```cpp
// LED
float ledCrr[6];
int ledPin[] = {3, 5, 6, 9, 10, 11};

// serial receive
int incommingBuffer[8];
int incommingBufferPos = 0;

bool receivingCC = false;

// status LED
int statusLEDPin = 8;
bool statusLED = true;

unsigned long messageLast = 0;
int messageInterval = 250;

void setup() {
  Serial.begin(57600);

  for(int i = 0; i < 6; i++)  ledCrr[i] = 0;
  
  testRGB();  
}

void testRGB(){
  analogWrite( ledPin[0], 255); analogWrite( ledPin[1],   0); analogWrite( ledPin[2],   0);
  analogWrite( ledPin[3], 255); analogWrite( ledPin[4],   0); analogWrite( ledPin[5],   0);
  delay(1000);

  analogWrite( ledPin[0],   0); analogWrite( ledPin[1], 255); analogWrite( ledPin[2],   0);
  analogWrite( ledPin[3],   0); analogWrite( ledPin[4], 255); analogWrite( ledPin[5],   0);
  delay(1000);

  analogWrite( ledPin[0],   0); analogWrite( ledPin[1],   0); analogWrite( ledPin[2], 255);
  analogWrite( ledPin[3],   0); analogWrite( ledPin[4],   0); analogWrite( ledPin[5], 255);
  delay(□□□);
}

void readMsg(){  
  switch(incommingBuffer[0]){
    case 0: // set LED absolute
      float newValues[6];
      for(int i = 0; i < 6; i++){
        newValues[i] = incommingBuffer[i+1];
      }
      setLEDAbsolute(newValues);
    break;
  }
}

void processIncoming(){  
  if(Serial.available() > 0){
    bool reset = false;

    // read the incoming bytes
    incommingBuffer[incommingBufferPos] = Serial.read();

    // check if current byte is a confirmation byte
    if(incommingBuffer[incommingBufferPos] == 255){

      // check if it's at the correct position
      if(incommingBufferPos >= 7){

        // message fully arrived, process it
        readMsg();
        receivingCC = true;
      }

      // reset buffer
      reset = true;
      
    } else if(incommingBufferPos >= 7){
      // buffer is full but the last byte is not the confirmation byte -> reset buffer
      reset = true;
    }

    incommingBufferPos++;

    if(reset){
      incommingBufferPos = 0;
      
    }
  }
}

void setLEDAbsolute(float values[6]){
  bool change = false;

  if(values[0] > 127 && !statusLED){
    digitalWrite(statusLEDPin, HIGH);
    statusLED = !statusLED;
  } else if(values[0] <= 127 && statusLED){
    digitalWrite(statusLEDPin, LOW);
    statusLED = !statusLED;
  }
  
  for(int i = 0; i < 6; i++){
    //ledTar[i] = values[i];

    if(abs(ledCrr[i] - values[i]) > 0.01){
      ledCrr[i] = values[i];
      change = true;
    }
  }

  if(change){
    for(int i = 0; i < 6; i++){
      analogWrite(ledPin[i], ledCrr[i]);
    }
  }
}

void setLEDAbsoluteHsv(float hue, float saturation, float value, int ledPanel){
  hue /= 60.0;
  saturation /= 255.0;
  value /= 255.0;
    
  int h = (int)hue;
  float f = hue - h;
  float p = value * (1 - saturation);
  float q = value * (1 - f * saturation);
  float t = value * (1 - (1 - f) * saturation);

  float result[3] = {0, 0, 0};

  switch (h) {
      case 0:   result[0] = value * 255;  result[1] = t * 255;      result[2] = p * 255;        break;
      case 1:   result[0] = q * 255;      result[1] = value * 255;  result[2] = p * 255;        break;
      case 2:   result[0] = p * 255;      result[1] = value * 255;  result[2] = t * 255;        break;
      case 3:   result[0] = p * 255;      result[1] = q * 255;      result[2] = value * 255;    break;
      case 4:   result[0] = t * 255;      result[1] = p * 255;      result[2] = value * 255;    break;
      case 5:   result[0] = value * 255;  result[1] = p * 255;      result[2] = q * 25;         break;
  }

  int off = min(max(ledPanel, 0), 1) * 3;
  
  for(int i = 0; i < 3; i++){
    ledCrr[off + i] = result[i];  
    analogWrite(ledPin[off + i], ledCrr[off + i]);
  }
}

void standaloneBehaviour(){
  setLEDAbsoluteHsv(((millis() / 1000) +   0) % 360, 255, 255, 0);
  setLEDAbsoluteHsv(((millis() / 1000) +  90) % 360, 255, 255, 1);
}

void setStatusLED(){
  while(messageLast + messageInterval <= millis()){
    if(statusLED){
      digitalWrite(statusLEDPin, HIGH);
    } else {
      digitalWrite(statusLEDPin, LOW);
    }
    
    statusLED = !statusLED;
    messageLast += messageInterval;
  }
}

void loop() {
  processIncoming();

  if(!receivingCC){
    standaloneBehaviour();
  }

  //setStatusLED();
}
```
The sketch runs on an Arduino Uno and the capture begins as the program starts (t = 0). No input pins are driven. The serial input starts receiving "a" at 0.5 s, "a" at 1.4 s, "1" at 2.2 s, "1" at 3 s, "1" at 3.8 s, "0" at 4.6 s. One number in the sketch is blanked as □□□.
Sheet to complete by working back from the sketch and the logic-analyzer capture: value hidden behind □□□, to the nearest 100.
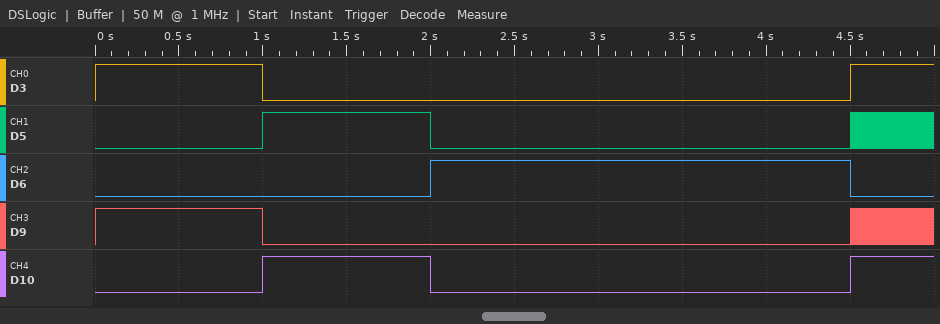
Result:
2500
